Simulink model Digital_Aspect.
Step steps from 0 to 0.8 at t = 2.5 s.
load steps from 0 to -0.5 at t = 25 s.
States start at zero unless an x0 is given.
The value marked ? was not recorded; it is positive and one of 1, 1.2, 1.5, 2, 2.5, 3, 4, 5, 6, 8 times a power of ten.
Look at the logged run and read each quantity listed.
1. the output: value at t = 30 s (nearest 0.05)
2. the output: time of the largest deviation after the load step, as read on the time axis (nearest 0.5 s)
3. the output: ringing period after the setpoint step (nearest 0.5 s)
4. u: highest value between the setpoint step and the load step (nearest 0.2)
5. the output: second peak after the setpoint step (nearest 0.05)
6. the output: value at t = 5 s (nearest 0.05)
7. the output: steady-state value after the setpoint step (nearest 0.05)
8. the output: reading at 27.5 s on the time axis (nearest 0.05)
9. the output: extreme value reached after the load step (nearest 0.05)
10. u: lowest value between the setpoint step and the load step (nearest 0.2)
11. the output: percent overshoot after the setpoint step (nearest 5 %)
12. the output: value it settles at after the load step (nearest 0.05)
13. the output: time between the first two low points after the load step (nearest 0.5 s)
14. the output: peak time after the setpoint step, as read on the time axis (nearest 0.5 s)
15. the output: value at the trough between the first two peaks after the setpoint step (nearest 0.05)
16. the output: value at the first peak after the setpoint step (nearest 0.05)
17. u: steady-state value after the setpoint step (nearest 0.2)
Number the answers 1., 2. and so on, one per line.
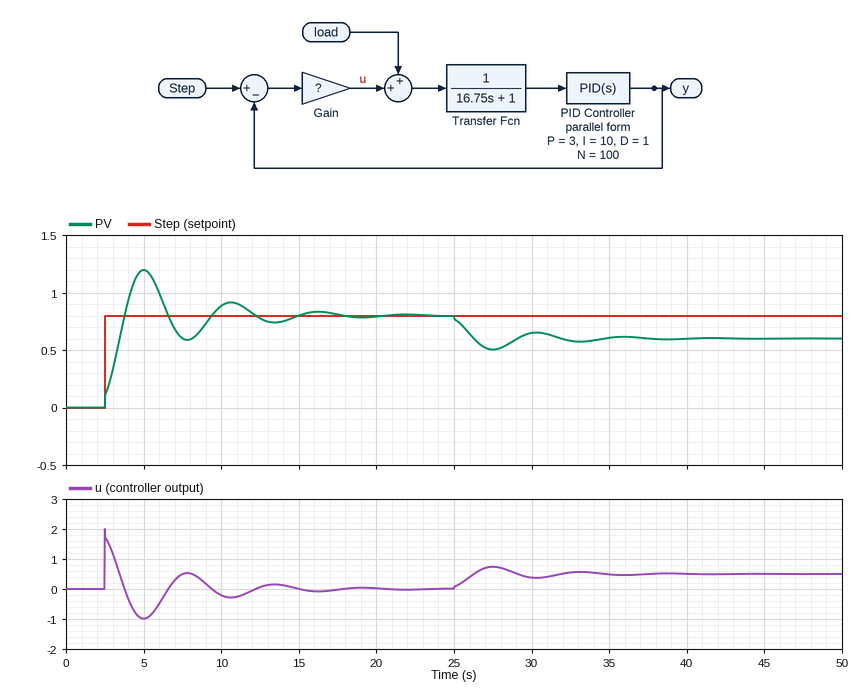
1. 0.65
2. 27.5 s
3. 5.5 s
4. 2.0
5. 0.90
6. 1.20
7. 0.80
8. 0.50
9. 0.50
10. -1.0
11. 50 %
12. 0.60
13. 5.5 s
14. 5.0 s
15. 0.60
16. 1.20
17. 0.0
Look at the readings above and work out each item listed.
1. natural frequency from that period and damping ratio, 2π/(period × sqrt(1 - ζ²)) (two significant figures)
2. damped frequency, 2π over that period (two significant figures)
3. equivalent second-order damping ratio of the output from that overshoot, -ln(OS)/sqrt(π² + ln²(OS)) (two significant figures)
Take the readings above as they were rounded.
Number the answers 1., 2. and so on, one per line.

1. 1.2 rad/s
2. 1.1 rad/s
3. 0.22
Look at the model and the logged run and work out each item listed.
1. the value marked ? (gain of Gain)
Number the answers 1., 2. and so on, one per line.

1. 2.5
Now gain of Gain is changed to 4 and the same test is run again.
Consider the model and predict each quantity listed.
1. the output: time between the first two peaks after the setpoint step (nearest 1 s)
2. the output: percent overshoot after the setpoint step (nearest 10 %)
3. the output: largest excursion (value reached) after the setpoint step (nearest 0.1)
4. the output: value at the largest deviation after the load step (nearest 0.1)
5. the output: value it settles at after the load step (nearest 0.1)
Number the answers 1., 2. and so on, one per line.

1. 5 s
2. 40 %
3. 1.1
4. 0.6
5. 0.7
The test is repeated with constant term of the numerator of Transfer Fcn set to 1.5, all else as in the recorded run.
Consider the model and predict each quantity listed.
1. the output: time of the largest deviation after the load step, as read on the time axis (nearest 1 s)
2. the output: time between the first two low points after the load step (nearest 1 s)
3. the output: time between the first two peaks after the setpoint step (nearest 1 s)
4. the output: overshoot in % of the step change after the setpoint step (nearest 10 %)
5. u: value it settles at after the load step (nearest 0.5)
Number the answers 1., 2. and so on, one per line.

1. 27 s
2. 5 s
3. 5 s
4. 40 %
5. 0.5
